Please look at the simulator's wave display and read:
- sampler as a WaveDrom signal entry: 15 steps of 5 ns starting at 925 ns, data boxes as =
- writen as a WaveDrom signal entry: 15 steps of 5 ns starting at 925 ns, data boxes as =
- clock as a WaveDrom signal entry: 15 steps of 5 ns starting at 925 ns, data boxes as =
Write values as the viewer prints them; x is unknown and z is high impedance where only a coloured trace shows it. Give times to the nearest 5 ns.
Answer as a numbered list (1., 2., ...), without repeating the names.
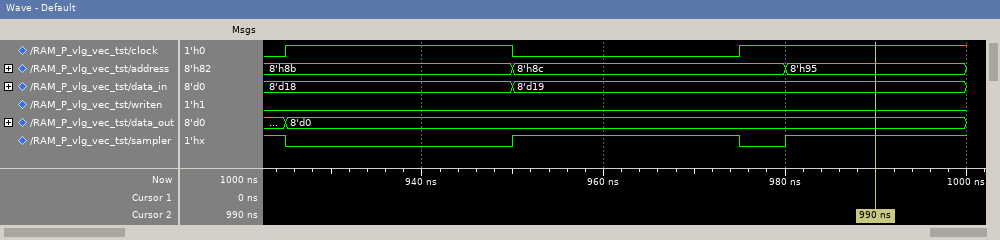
1. {name: 'sampler', wave: '0....1....01...'}
2. {name: 'writen', wave: '0..............'}
3. {name: 'clock', wave: '1....0....1....'}
